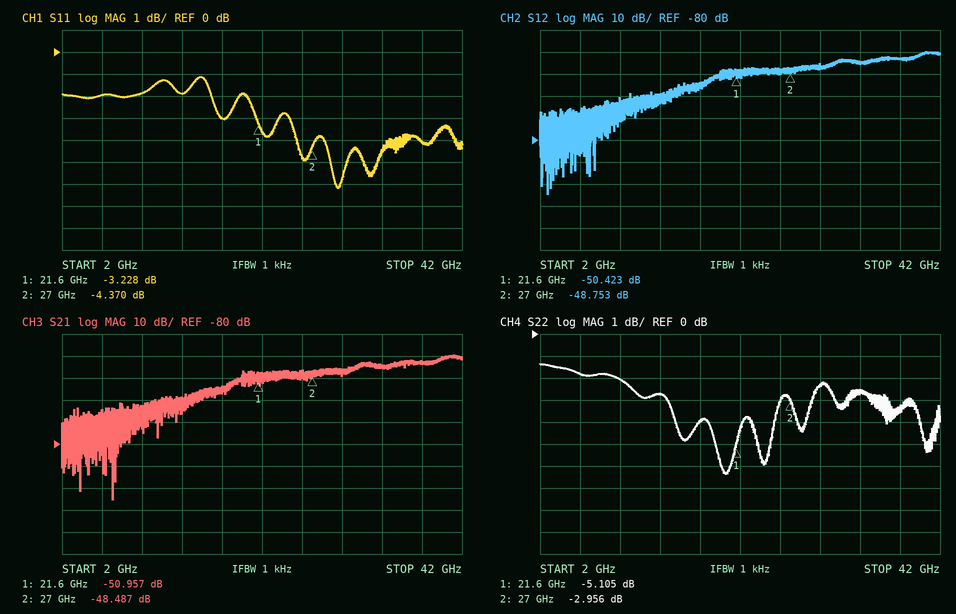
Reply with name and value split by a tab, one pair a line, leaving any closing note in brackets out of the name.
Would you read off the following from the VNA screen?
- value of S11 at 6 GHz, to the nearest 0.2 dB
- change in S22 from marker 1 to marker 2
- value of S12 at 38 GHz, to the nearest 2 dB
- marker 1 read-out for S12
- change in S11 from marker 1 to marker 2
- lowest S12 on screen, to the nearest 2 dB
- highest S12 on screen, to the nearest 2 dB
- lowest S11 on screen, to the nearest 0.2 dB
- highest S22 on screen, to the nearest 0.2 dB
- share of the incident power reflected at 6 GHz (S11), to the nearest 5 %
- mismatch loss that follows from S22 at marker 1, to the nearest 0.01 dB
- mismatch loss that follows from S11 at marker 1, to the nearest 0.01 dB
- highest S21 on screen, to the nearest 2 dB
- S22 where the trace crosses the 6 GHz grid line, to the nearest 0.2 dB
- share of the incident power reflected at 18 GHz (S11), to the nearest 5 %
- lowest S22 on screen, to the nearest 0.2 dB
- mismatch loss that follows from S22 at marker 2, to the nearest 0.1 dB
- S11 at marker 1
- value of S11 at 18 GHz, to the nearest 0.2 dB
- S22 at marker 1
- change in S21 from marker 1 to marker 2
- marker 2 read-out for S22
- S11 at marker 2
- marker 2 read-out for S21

value of S11 at 6 GHz, to the nearest 0.2 dB	-2.0 dB
change in S22 from marker 1 to marker 2	2.149 dB
value of S12 at 38 GHz, to the nearest 2 dB	-44 dB
marker 1 read-out for S12	-50.423 dB
change in S11 from marker 1 to marker 2	-1.142 dB
lowest S12 on screen, to the nearest 2 dB	-104 dB
highest S12 on screen, to the nearest 2 dB	-40 dB
lowest S11 on screen, to the nearest 0.2 dB	-6.2 dB
highest S22 on screen, to the nearest 0.2 dB	-1.4 dB
share of the incident power reflected at 6 GHz (S11), to the nearest 5 %	65 %
mismatch loss that follows from S22 at marker 1, to the nearest 0.01 dB	1.60 dB
mismatch loss that follows from S11 at marker 1, to the nearest 0.01 dB	2.80 dB
highest S21 on screen, to the nearest 2 dB	-40 dB
S22 where the trace crosses the 6 GHz grid line, to the nearest 0.2 dB	-1.8 dB
share of the incident power reflected at 18 GHz (S11), to the nearest 5 %	50 %
lowest S22 on screen, to the nearest 0.2 dB	-6.4 dB
mismatch loss that follows from S22 at marker 2, to the nearest 0.1 dB	3.1 dB
S11 at marker 1	-3.228 dB
value of S11 at 18 GHz, to the nearest 0.2 dB	-3.0 dB
S22 at marker 1	-5.105 dB
change in S21 from marker 1 to marker 2	2.470 dB
marker 2 read-out for S22	-2.956 dB
S11 at marker 2	-4.370 dB
marker 2 read-out for S21	-48.487 dB
